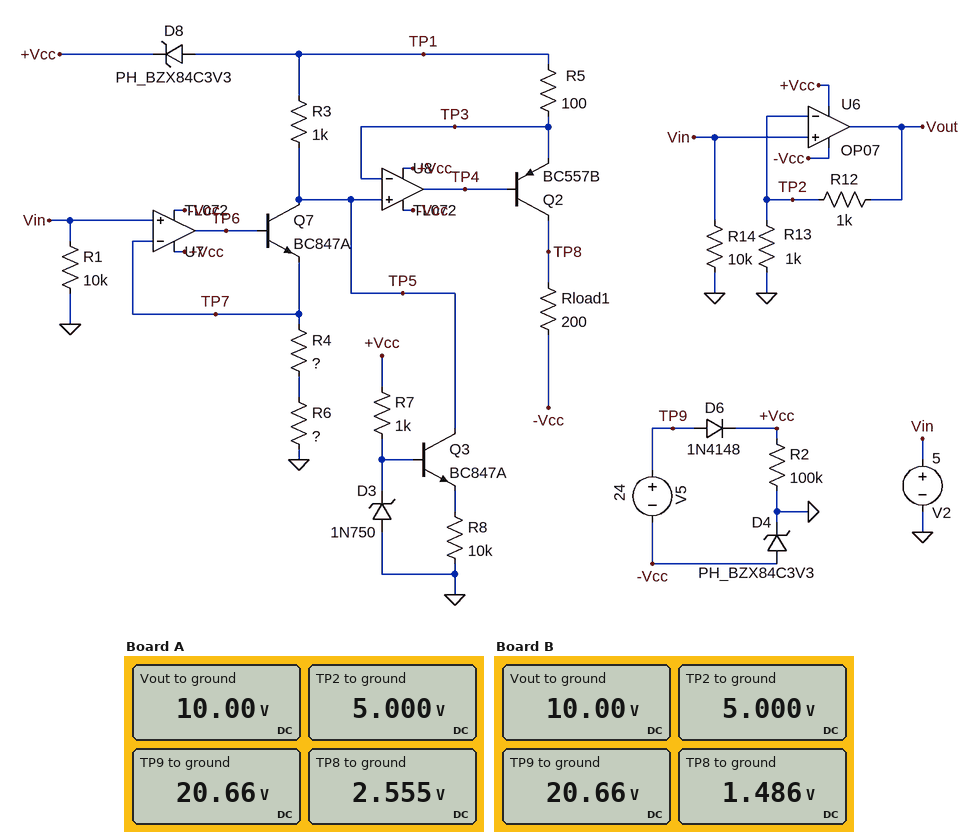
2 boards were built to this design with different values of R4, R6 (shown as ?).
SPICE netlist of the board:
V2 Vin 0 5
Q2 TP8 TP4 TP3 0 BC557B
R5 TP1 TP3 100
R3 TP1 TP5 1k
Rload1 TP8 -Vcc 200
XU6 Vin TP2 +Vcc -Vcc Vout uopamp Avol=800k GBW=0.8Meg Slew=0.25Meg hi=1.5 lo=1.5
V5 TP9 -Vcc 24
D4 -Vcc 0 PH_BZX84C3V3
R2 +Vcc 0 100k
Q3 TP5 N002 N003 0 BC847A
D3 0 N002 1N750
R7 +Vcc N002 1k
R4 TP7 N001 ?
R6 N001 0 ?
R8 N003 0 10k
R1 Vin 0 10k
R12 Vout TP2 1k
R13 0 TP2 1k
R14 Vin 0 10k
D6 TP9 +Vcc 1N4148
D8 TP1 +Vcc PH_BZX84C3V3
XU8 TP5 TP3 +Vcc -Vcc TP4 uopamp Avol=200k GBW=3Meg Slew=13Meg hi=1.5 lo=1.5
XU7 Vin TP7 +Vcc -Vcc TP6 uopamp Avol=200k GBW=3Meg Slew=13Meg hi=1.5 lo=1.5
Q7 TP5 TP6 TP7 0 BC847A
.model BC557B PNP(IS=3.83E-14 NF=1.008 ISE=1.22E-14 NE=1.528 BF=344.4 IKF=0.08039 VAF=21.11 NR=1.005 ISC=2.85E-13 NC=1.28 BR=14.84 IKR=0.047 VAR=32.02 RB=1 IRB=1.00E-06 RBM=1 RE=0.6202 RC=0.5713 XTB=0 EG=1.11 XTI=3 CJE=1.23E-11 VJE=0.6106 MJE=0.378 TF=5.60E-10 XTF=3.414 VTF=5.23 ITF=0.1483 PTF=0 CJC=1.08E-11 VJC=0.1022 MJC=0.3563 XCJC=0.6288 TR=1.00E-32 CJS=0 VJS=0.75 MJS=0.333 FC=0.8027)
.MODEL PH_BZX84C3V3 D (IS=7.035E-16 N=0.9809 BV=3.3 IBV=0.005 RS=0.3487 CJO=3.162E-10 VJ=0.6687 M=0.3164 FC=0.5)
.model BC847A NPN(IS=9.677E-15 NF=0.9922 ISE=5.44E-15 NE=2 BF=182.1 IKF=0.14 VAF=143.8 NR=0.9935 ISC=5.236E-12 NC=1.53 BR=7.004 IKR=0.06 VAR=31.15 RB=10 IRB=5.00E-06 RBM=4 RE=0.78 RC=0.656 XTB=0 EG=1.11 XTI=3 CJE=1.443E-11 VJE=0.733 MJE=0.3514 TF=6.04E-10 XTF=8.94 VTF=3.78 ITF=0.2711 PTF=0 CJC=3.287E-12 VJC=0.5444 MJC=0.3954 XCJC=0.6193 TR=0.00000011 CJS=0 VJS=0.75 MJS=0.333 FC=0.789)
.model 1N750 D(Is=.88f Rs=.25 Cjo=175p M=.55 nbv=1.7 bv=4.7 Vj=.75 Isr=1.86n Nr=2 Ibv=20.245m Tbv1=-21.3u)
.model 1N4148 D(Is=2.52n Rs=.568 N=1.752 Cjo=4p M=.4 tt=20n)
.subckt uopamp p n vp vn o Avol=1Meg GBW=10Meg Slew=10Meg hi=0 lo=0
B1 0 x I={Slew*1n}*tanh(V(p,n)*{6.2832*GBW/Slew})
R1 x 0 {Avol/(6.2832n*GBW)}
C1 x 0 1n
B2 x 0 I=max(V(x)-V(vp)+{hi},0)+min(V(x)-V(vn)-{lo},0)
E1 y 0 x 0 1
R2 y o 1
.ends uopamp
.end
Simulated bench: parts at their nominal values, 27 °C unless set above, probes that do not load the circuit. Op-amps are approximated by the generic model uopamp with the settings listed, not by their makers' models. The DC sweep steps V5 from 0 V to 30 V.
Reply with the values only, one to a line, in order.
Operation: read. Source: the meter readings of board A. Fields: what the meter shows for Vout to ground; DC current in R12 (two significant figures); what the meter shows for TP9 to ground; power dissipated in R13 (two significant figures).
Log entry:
10.00 V
5.0 mA
20.66 V
25 mW
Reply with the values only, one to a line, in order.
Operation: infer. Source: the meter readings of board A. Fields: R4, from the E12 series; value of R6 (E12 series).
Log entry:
1.8 kΩ
150 Ω
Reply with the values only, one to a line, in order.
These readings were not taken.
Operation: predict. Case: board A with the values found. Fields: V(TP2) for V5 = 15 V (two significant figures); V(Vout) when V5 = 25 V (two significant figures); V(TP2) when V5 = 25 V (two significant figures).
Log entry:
4.7 V
10 V
5.0 V
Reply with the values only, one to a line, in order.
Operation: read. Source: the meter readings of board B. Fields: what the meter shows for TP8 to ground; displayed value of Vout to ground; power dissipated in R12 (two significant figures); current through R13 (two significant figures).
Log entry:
1.486 V
10.00 V
25 mW
5.0 mA
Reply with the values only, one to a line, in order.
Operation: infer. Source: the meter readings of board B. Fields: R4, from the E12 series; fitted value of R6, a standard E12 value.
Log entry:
2.2 kΩ
270 Ω
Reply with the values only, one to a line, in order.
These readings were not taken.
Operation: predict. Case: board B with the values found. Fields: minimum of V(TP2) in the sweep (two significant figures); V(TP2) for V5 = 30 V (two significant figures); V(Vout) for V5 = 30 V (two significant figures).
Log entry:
-430 mV
5.0 V
10 V
